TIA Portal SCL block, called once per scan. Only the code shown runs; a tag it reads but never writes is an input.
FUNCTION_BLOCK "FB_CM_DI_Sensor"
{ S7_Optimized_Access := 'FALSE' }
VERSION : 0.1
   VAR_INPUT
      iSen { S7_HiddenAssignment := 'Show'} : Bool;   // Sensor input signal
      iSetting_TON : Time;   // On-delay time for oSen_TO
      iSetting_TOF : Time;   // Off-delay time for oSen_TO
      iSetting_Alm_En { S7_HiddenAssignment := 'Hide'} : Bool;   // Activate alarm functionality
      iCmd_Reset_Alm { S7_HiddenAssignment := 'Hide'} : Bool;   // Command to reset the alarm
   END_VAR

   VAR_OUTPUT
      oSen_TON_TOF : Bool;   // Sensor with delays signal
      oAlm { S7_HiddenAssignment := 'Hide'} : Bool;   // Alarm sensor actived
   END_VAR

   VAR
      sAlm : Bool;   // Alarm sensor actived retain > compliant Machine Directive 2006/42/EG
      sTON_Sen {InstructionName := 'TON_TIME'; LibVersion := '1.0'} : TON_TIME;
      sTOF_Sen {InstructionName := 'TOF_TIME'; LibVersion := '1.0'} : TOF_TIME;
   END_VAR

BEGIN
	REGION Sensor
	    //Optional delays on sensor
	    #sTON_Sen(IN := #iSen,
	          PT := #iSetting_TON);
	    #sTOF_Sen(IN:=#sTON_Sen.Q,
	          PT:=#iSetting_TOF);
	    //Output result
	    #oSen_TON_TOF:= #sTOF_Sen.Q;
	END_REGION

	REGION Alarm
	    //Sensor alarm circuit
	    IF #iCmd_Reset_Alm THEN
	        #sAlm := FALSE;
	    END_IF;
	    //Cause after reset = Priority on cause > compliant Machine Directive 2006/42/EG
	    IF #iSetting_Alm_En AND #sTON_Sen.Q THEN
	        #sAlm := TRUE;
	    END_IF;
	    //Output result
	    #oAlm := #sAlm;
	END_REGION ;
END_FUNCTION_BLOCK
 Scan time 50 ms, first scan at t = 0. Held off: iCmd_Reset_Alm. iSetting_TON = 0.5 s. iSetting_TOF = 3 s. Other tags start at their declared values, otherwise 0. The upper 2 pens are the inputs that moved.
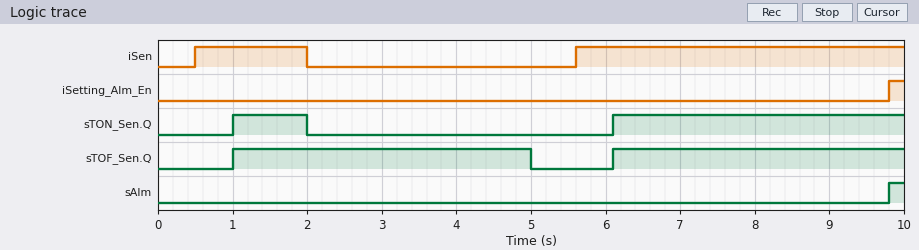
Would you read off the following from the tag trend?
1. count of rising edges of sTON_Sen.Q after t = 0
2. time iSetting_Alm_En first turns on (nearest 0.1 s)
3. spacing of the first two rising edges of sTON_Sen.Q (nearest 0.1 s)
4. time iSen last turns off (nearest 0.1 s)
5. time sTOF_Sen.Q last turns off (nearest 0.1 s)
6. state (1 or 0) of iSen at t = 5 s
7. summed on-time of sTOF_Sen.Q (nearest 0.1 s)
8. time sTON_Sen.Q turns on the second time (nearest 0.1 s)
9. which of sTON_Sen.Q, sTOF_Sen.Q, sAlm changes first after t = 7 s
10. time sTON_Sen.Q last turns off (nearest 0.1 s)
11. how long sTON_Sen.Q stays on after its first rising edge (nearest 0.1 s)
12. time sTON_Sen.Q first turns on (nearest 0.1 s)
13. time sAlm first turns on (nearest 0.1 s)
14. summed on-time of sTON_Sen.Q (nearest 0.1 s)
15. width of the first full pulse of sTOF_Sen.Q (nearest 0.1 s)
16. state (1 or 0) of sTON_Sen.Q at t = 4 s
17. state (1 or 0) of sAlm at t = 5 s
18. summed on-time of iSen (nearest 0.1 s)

2
9.8 s
5.1 s
2.0 s
5.0 s
0
7.9 s
6.1 s
sAlm
2.0 s
1.0 s
1.0 s
9.8 s
4.9 s
4.0 s
0
0
5.9 s
